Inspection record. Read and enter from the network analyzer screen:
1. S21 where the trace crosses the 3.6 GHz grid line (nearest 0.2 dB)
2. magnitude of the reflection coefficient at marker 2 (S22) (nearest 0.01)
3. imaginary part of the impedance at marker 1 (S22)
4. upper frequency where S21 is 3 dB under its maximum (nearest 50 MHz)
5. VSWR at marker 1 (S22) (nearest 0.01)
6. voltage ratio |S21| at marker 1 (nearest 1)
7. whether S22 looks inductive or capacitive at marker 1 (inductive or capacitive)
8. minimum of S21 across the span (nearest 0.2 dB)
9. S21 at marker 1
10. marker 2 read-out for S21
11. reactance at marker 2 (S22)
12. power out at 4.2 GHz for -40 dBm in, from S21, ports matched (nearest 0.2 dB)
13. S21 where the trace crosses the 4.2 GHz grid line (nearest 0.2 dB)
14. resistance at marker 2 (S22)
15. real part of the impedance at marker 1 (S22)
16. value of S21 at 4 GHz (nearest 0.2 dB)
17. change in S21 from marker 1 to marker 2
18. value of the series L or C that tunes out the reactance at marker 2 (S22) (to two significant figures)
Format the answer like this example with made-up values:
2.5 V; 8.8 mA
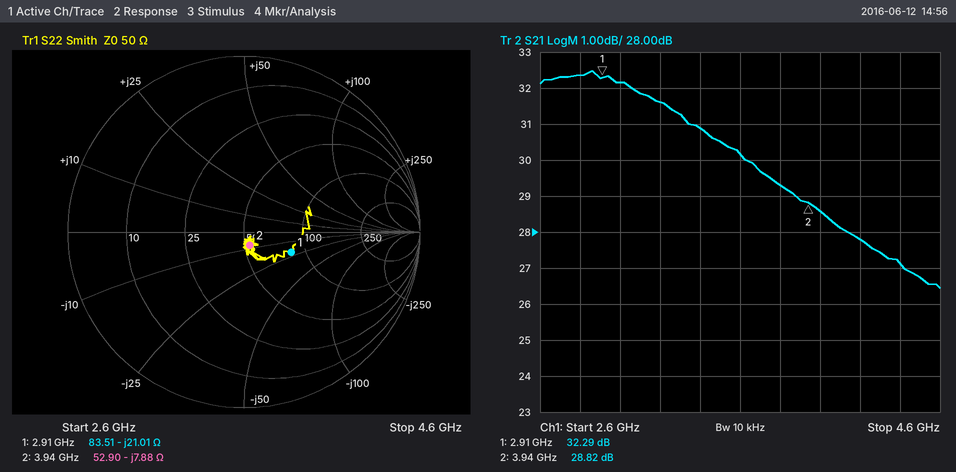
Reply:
30.2 dB; 0.08; -21.01 Ω; 3.75 GHz; 1.83; 41; capacitive; 26.4 dB; 32.29 dB; 28.82 dB; -7.88 Ω; -12.2 dBm; 27.8 dB; 52.90 Ω; 83.51 Ω; 28.6 dB; -3.47 dB; 320 pH
